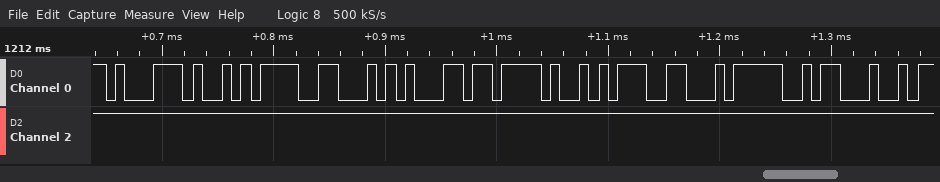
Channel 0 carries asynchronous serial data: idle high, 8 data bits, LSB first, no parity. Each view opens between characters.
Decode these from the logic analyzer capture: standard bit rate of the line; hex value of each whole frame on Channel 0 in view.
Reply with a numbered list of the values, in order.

1. 115200 baud
2. 71, EA, 46, B1, 2F, 9D, F4, 1A
